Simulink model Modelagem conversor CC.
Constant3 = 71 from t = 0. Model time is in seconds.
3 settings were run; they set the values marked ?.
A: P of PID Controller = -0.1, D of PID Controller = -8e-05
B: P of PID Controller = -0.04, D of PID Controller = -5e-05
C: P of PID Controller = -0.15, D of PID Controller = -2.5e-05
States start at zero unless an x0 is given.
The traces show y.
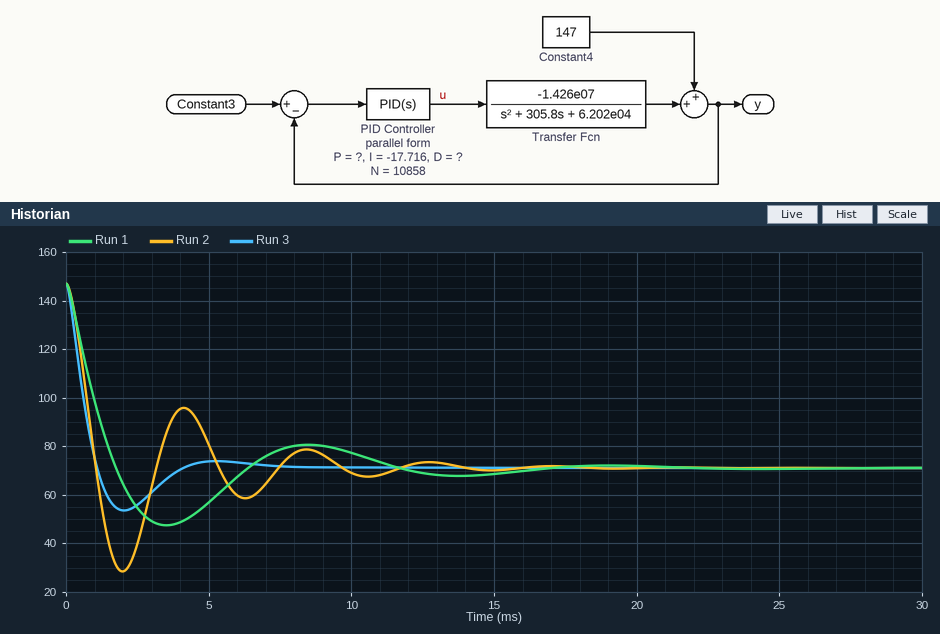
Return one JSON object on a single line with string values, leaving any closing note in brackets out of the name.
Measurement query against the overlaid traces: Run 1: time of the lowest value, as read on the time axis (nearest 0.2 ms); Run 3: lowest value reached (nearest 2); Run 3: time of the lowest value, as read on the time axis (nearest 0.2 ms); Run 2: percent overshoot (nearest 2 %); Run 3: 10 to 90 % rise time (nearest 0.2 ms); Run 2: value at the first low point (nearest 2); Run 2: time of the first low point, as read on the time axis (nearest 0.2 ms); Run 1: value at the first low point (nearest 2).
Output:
{"Run 1: time of the lowest value, as read on the time axis": "3.6 ms", "Run 3: lowest value reached": "54", "Run 3: time of the lowest value, as read on the time axis": "2.0 ms", "Run 2: percent overshoot": "56 %", "Run 3: 10 to 90 % rise time": "0.8 ms", "Run 2: value at the first low point": "28", "Run 2: time of the first low point, as read on the time axis": "2.0 ms", "Run 1: value at the first low point": "48"}
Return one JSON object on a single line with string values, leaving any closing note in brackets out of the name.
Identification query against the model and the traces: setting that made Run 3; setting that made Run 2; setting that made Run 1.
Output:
{"setting that made Run 3": "A", "setting that made Run 2": "C", "setting that made Run 1": "B"}
